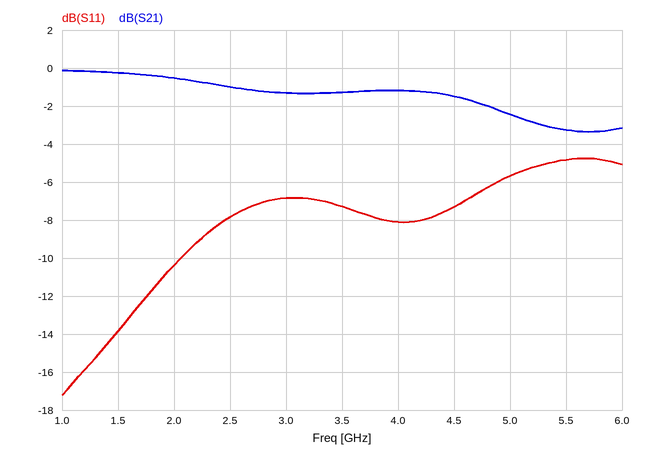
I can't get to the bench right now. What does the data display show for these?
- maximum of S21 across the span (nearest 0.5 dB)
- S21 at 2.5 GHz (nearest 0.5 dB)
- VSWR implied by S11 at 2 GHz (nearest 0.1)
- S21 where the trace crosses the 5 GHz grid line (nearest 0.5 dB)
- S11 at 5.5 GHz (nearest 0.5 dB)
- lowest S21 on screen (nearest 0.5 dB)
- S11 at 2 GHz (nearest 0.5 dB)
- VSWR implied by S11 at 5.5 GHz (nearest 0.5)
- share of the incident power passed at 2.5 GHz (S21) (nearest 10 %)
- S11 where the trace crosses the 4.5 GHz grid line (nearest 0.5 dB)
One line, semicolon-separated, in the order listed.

0.0 dB; -1.0 dB; 1.9; -2.5 dB; -5.0 dB; -3.5 dB; -10.5 dB; 3.5; 80 %; -7.5 dB
